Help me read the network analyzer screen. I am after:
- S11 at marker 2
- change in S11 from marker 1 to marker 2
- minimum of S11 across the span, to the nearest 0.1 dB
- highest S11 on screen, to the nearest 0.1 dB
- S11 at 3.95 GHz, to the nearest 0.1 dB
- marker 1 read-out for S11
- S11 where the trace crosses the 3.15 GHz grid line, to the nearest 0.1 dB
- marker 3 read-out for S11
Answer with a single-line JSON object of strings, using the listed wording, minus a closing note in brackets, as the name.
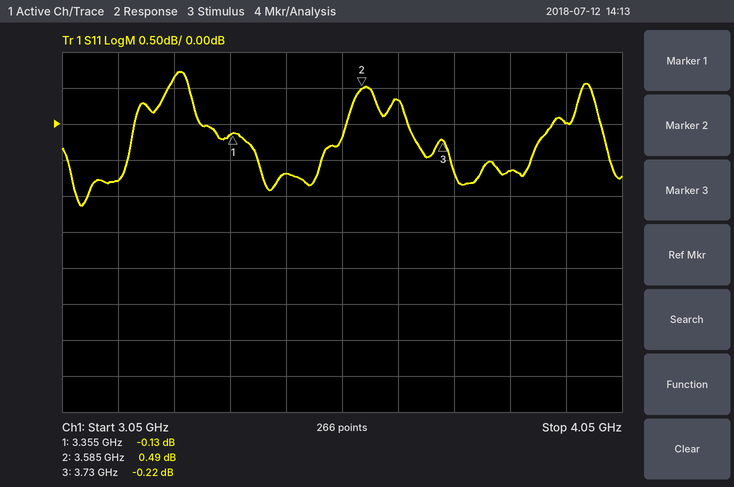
{"S11 at marker 2": "0.49 dB", "change in S11 from marker 1 to marker 2": "0.62 dB", "minimum of S11 across the span, to the nearest 0.1 dB": "-1.1 dB", "highest S11 on screen, to the nearest 0.1 dB": "0.7 dB", "S11 at 3.95 GHz, to the nearest 0.1 dB": "0.0 dB", "marker 1 read-out for S11": "-0.13 dB", "S11 where the trace crosses the 3.15 GHz grid line, to the nearest 0.1 dB": "-0.8 dB", "marker 3 read-out for S11": "-0.22 dB"}
